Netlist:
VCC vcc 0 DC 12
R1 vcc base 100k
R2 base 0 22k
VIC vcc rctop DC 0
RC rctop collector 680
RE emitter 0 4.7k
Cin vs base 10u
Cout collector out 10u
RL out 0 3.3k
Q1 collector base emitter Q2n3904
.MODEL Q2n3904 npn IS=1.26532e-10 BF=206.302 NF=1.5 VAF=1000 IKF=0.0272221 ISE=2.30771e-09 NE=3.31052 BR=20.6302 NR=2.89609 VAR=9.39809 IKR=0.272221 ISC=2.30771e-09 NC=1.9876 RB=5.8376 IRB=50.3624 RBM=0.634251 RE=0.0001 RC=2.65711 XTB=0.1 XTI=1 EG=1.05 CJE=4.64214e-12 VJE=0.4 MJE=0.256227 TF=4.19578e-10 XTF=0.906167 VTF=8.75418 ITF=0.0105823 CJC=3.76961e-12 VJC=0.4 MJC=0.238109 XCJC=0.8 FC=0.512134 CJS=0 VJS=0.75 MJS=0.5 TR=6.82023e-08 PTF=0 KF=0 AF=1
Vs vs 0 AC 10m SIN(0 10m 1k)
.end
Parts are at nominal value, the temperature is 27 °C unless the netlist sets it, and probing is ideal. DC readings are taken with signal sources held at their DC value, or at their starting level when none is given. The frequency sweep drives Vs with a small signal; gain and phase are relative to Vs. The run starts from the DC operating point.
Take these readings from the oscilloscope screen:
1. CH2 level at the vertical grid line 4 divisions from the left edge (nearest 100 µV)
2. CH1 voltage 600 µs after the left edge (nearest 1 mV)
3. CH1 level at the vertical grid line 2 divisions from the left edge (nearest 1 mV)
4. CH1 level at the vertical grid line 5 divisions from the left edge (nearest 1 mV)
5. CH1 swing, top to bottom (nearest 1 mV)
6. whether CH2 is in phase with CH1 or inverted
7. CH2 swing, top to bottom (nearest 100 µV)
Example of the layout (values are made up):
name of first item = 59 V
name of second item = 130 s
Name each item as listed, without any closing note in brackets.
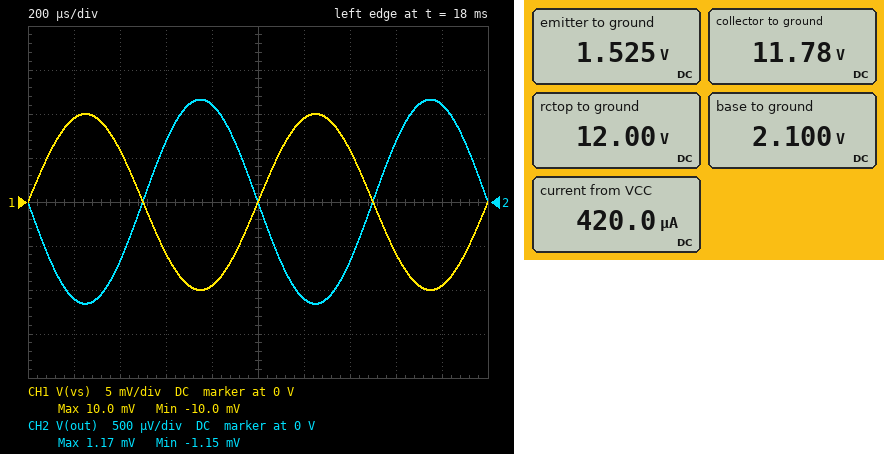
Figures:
CH2 level at the vertical grid line 4 divisions from the left edge = 1.1 mV
CH1 voltage 600 µs after the left edge = -6 mV
CH1 level at the vertical grid line 2 divisions from the left edge = 6 mV
CH1 level at the vertical grid line 5 divisions from the left edge = 0 V
CH1 swing, top to bottom = 20 mV
whether CH2 is in phase with CH1 or inverted = inverted
CH2 swing, top to bottom = 2.3 mV
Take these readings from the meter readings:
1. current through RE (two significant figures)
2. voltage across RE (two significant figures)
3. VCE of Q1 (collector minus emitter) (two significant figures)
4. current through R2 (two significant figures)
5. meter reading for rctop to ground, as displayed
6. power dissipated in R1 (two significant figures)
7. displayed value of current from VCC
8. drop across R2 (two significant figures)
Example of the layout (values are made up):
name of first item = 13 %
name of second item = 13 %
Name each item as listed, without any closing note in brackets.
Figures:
current through RE = 320 µA
voltage across RE = 1.5 V
VCE of Q1 (collector minus emitter) = 10 V
current through R2 = 95 µA
meter reading for rctop to ground, as displayed = 12.00 V
power dissipated in R1 = 980 µW
displayed value of current from VCC = 420.0 µA
drop across R2 = 2.1 V
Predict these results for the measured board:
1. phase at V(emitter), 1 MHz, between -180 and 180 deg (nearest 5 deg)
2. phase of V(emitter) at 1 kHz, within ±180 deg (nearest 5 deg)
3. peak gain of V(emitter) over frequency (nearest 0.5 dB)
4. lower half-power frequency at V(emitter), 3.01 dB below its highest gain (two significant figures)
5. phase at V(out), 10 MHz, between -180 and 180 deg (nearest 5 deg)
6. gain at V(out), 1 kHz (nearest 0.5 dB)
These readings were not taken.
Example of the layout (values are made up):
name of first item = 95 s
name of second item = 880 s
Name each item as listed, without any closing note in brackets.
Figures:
phase at V(emitter), 1 MHz, between -180 and 180 deg = 0 deg
phase of V(emitter) at 1 kHz, within ±180 deg = 0 deg
peak gain of V(emitter) over frequency = 0 dB
lower half-power frequency at V(emitter), 3.01 dB below its highest gain = 940 mHz
phase at V(out), 10 MHz, between -180 and 180 deg = 145 deg
gain at V(out), 1 kHz = -18.5 dB
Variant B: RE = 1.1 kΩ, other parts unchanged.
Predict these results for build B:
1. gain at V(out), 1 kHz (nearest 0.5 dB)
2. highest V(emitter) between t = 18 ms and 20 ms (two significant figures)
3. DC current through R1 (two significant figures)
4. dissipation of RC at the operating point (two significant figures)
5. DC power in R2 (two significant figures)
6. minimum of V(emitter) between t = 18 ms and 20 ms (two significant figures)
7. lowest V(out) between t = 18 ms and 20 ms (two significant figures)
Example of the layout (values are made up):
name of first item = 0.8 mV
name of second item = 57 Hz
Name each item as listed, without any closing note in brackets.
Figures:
gain at V(out), 1 kHz = -6.0 dB
highest V(emitter) between t = 18 ms and 20 ms = 1.4 V
DC current through R1 = 100 µA
dissipation of RC at the operating point = 1.0 mW
DC power in R2 = 180 µW
minimum of V(emitter) between t = 18 ms and 20 ms = 1.3 V
lowest V(out) between t = 18 ms and 20 ms = -4.9 mV
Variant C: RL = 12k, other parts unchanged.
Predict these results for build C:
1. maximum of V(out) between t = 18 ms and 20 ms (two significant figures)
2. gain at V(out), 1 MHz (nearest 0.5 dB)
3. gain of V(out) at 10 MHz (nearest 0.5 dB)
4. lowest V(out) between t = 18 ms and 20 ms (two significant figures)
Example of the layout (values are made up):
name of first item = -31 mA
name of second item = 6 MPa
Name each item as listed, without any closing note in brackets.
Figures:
maximum of V(out) between t = 18 ms and 20 ms = 1.3 mV
gain at V(out), 1 MHz = -17.5 dB
gain of V(out) at 10 MHz = -16.0 dB
lowest V(out) between t = 18 ms and 20 ms = -1.3 mV
